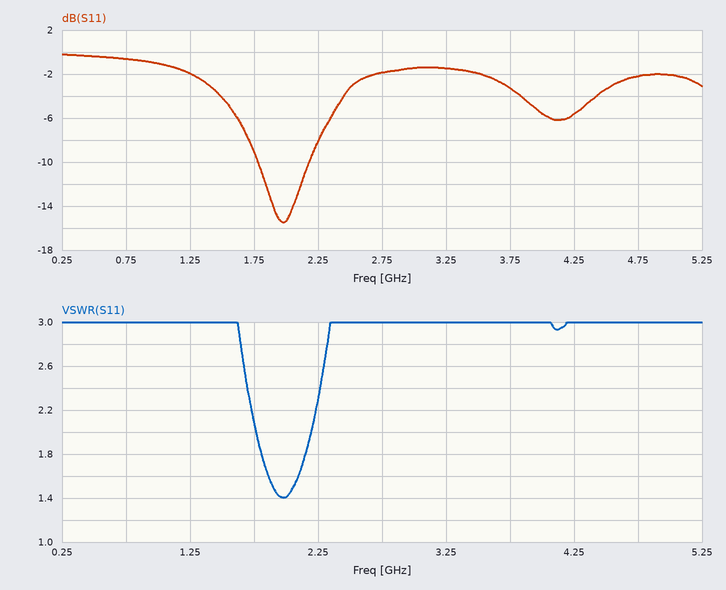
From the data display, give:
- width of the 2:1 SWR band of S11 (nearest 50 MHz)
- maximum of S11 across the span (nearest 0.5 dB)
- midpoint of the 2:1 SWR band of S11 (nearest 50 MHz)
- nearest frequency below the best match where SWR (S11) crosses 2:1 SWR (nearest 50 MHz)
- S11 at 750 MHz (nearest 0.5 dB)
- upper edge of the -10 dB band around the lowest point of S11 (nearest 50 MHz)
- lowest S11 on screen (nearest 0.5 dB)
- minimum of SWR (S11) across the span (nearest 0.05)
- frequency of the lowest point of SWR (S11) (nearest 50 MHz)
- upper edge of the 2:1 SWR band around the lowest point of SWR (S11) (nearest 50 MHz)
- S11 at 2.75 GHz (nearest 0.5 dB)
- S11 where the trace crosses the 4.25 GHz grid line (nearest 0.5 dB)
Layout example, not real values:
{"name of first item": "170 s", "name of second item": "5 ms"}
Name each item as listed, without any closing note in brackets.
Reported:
{"width of the 2:1 SWR band of S11": "450 MHz", "maximum of S11 across the span": "0.0 dB", "midpoint of the 2:1 SWR band of S11": "2.00 GHz", "nearest frequency below the best match where SWR (S11) crosses 2:1 SWR": "1.75 GHz", "S11 at 750 MHz": "-0.5 dB", "upper edge of the -10 dB band around the lowest point of S11": "2.20 GHz", "lowest S11 on screen": "-15.5 dB", "minimum of SWR (S11) across the span": "1.40", "frequency of the lowest point of SWR (S11)": "2.00 GHz", "upper edge of the 2:1 SWR band around the lowest point of SWR (S11)": "2.20 GHz", "S11 at 2.75 GHz": "-2.0 dB", "S11 where the trace crosses the 4.25 GHz grid line": "-5.5 dB"}
